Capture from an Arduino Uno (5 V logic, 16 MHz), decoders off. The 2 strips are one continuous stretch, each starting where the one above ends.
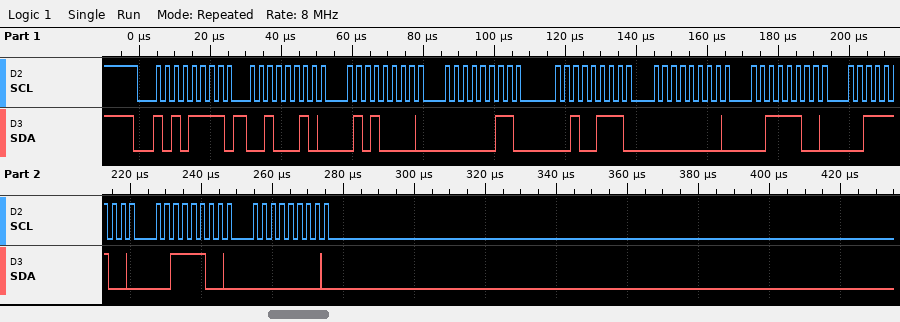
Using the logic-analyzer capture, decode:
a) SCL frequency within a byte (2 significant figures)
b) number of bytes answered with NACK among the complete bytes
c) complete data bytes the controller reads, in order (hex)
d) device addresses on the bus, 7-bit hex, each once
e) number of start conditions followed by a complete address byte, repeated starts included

400 kHz
0
22 50 03 27 00 3C 3C 3C 00
0x57
1
